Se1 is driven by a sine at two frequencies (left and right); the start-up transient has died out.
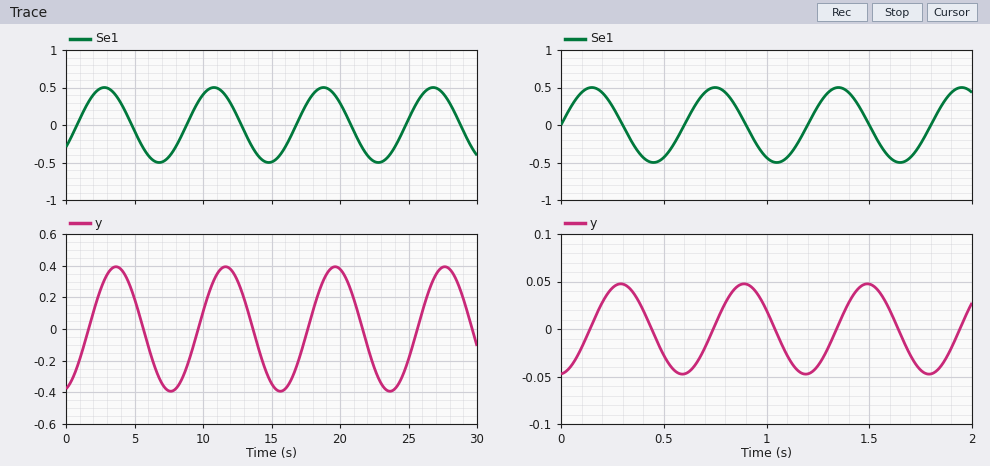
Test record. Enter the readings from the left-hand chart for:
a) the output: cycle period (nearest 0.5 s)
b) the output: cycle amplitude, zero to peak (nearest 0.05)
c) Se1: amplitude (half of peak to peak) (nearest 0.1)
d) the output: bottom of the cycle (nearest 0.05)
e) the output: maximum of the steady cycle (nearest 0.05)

8.0 s
0.40
0.5
-0.40
0.40
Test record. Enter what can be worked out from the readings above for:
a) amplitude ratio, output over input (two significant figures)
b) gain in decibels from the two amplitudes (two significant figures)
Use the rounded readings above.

0.80
-1.9 dB
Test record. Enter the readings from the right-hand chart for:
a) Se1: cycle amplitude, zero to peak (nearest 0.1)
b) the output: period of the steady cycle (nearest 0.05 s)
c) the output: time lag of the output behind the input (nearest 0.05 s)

0.5
0.60 s
0.15 s
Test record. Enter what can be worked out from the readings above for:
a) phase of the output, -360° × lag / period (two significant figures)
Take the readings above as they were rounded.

-90°
